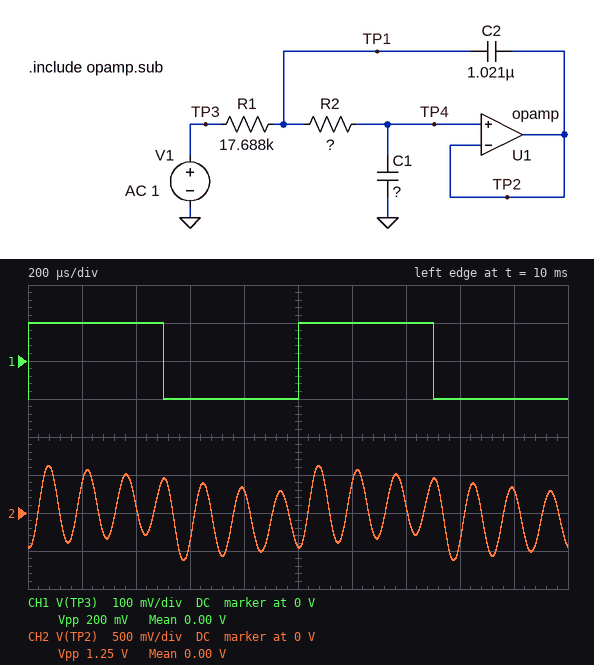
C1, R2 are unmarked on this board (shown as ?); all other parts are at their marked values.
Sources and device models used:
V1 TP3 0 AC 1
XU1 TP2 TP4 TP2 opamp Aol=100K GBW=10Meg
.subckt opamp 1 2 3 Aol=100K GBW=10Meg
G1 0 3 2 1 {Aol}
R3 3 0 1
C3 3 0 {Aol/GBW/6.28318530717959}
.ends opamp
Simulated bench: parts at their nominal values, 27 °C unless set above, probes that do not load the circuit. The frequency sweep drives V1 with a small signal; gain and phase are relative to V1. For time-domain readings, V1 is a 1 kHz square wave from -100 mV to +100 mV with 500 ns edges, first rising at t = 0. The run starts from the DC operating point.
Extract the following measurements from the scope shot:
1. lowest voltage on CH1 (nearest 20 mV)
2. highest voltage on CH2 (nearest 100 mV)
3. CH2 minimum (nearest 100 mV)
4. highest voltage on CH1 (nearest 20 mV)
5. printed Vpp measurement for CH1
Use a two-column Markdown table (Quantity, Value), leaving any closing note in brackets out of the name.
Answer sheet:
| Quantity | Value |
|---|---|
| lowest voltage on CH1 | -100 mV |
| highest voltage on CH2 | 600 mV |
| CH2 minimum | -600 mV |
| highest voltage on CH1 | 100 mV |
| printed Vpp measurement for CH1 | 200 mV |
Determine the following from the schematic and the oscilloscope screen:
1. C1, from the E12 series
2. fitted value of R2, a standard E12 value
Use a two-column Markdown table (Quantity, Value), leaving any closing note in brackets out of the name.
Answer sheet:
| Quantity | Value |
|---|---|
| C1, from the E12 series | 39 pF |
| fitted value of R2, a standard E12 value | 330 Ω |
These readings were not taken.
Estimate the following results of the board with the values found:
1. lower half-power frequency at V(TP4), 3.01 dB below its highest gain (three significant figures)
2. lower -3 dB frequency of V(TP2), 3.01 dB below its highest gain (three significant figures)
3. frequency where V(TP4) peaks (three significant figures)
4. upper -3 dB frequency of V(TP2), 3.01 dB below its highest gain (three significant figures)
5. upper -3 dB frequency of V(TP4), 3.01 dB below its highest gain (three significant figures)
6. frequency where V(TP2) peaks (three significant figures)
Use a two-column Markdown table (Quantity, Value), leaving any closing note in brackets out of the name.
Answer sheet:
| Quantity | Value |
|---|---|
| lower half-power frequency at V(TP4), 3.01 dB below its highest gain | 6.84 kHz |
| lower -3 dB frequency of V(TP2), 3.01 dB below its highest gain | 6.84 kHz |
| frequency where V(TP4) peaks | 6.98 kHz |
| upper -3 dB frequency of V(TP2), 3.01 dB below its highest gain | 7.11 kHz |
| upper -3 dB frequency of V(TP4), 3.01 dB below its highest gain | 7.11 kHz |
| frequency where V(TP2) peaks | 6.98 kHz |
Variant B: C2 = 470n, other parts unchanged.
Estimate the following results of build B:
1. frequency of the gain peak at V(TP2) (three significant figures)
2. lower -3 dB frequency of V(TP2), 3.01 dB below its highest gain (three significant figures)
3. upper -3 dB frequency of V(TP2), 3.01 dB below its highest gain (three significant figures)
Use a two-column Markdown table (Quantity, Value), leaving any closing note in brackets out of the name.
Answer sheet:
| Quantity | Value |
|---|---|
| frequency of the gain peak at V(TP2) | 10.3 kHz |
| lower -3 dB frequency of V(TP2), 3.01 dB below its highest gain | 10.0 kHz |
| upper -3 dB frequency of V(TP2), 3.01 dB below its highest gain | 10.5 kHz |
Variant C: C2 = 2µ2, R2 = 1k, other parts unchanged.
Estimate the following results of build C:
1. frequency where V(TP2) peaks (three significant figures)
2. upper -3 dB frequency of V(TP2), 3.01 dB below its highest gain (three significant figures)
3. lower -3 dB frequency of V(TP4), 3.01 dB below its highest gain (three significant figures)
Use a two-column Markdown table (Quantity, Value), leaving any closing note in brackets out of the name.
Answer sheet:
| Quantity | Value |
|---|---|
| frequency where V(TP2) peaks | 3.44 kHz |
| upper -3 dB frequency of V(TP2), 3.01 dB below its highest gain | 3.48 kHz |
| lower -3 dB frequency of V(TP4), 3.01 dB below its highest gain | 3.40 kHz |
